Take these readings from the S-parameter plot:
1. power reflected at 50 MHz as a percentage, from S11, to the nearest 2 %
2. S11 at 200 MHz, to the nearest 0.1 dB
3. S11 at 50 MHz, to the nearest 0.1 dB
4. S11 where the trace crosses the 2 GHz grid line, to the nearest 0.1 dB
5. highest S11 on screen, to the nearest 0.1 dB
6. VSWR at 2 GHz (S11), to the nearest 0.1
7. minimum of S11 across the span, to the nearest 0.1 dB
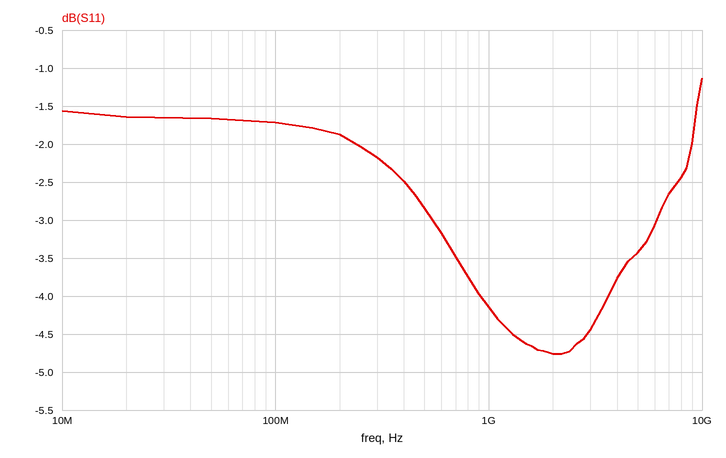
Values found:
68 %
-1.9 dB
-1.7 dB
-4.8 dB
-1.1 dB
3.7
-4.8 dB
